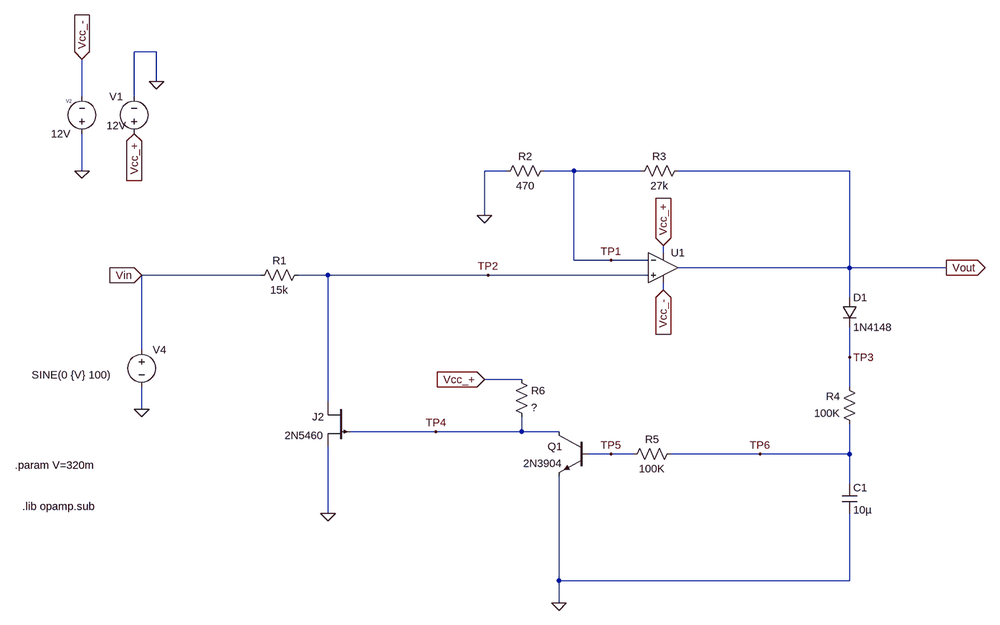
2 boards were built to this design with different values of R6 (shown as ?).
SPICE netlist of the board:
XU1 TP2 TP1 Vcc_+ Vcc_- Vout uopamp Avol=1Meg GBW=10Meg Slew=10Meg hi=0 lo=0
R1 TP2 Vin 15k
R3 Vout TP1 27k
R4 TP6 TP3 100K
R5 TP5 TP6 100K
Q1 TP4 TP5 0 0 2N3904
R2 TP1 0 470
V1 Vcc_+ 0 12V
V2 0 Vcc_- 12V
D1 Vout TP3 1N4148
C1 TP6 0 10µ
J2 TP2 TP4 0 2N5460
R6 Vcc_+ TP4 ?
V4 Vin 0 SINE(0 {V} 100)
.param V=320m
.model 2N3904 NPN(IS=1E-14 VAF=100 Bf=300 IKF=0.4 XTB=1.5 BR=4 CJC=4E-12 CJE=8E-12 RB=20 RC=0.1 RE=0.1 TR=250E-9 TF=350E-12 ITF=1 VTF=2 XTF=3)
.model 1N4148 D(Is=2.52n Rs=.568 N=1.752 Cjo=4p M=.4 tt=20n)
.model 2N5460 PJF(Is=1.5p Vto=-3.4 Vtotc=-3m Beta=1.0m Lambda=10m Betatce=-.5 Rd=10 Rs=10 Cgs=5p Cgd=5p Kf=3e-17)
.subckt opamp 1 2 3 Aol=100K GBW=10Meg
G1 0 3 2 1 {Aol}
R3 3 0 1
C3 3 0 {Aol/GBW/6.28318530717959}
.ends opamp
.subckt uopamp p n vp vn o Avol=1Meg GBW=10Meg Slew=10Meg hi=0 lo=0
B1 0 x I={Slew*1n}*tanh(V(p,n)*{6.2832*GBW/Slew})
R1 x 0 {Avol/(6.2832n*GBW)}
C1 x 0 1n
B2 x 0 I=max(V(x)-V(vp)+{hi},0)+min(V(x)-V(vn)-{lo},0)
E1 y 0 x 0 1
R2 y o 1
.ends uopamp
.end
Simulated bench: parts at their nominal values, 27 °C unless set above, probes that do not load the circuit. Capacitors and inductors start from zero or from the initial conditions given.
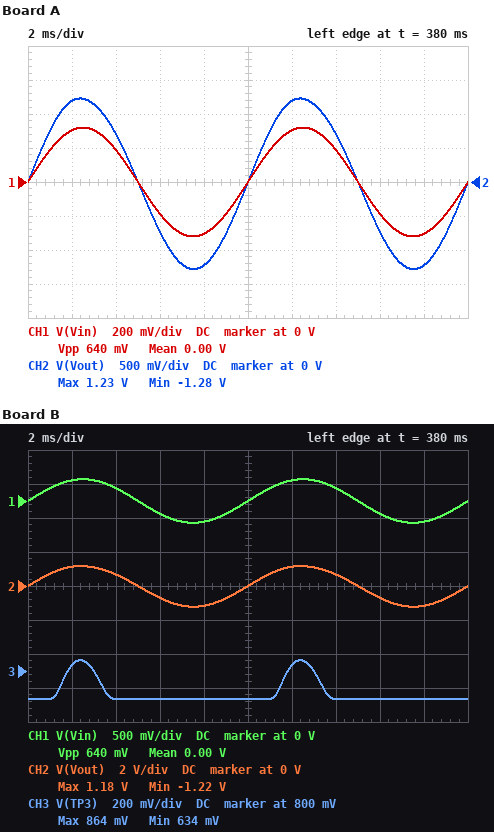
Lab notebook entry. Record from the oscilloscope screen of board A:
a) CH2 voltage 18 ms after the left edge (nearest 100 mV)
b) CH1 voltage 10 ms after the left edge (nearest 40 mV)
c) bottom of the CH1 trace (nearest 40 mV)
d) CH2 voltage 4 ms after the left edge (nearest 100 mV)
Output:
-1.2 V
0 V
-320 mV
700 mV
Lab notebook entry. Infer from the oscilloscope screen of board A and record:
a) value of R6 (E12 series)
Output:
68 kΩ
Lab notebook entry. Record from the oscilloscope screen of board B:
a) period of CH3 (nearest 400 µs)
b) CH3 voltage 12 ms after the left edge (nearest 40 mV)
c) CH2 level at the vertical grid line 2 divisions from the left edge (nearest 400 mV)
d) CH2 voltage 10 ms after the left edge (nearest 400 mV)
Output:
10.0 ms
840 mV
800 mV
0 V
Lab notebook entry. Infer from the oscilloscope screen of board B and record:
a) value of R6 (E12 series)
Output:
82 kΩ
